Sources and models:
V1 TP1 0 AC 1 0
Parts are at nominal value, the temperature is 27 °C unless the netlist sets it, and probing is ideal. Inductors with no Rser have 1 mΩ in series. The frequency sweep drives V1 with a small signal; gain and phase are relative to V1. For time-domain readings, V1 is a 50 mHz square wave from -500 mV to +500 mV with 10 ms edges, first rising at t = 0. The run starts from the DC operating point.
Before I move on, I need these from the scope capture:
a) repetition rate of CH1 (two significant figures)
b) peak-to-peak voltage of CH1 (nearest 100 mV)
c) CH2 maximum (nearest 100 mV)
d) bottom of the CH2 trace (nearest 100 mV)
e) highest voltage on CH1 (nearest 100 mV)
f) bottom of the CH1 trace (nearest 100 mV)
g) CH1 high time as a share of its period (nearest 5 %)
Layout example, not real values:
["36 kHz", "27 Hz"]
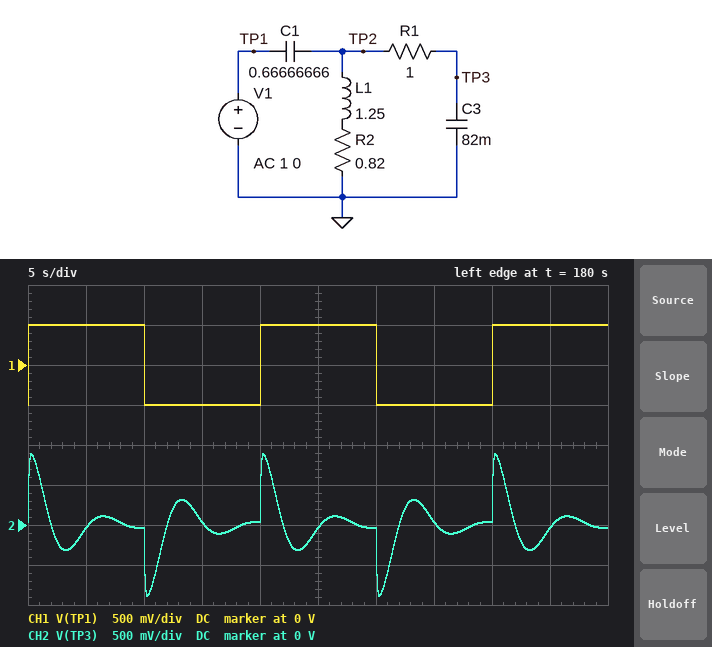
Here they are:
["50 mHz", "1.0 V", "900 mV", "-900 mV", "500 mV", "-500 mV", "50 %"]
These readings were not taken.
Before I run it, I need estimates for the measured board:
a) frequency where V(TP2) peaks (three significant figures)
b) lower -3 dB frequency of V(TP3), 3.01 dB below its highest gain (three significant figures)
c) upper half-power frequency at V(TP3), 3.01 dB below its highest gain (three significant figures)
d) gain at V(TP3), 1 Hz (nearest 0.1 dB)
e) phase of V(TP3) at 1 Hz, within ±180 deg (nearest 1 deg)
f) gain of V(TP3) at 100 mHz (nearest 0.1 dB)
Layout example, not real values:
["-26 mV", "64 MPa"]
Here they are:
["179 mHz", "133 mHz", "303 mHz", "-1.6 dB", "-24 deg", "-3.9 dB"]
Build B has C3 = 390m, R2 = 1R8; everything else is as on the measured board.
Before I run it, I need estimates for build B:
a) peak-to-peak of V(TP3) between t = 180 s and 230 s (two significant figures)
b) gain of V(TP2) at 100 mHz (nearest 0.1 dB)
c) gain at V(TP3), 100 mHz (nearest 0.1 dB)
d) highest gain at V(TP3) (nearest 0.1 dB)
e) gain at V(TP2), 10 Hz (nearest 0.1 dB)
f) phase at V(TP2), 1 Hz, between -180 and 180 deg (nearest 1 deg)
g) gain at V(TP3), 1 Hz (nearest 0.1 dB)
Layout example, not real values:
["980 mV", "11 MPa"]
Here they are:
["1.1 V", "-4.3 dB", "-4.6 dB", "-3.2 dB", "0 dB", "11 deg", "-9.1 dB"]
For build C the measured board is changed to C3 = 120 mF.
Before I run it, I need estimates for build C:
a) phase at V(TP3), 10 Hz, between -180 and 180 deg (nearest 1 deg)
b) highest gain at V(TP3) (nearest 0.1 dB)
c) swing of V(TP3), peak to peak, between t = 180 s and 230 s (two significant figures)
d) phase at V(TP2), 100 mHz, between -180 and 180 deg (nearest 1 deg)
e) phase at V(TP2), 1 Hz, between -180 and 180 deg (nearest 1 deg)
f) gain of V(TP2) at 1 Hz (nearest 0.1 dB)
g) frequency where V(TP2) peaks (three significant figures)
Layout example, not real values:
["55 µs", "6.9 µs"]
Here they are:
["-81 deg", "3.8 dB", "1.6 V", "100 deg", "5 deg", "-0.7 dB", "176 mHz"]
